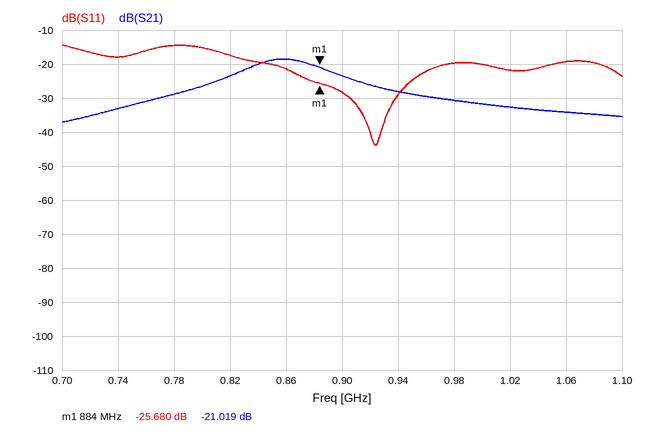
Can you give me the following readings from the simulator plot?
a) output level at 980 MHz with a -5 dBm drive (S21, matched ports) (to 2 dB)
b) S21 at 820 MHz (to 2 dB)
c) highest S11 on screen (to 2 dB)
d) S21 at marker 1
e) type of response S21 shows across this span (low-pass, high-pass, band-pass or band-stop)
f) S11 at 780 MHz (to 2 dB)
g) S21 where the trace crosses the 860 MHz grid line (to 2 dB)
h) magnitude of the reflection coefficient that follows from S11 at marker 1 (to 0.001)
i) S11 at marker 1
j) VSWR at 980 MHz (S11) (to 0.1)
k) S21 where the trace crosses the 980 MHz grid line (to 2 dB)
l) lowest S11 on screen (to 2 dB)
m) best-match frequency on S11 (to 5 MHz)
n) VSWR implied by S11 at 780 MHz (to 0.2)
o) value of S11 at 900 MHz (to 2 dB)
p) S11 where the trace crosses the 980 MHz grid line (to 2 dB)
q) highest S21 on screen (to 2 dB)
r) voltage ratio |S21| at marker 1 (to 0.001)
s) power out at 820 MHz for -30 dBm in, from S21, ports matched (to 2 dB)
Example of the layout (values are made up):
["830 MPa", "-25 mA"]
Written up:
["-36 dBm", "-24 dB", "-14 dB", "-21.019 dB", "band-pass", "-14 dB", "-18 dB", "0.052", "-25.680 dB", "1.2", "-30 dB", "-44 dB", "925 MHz", "1.4", "-28 dB", "-20 dB", "-18 dB", "0.089", "-54 dBm"]
